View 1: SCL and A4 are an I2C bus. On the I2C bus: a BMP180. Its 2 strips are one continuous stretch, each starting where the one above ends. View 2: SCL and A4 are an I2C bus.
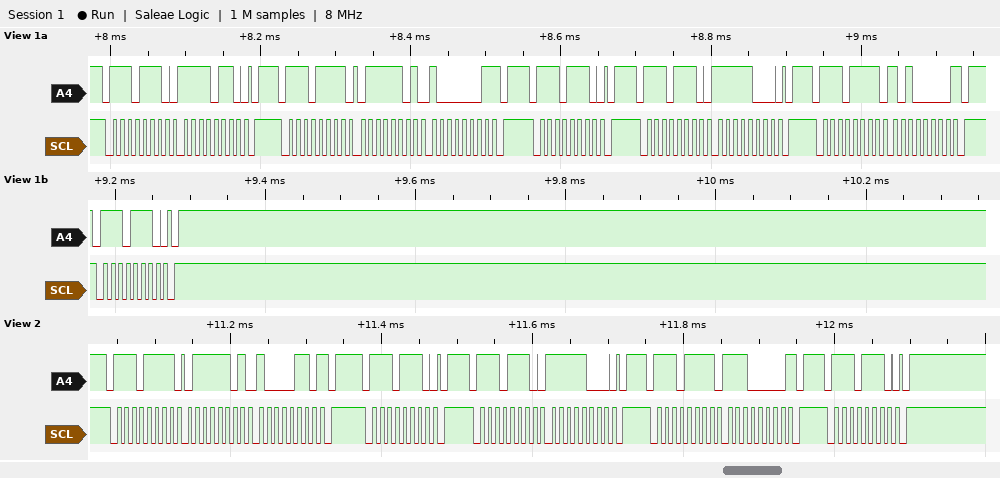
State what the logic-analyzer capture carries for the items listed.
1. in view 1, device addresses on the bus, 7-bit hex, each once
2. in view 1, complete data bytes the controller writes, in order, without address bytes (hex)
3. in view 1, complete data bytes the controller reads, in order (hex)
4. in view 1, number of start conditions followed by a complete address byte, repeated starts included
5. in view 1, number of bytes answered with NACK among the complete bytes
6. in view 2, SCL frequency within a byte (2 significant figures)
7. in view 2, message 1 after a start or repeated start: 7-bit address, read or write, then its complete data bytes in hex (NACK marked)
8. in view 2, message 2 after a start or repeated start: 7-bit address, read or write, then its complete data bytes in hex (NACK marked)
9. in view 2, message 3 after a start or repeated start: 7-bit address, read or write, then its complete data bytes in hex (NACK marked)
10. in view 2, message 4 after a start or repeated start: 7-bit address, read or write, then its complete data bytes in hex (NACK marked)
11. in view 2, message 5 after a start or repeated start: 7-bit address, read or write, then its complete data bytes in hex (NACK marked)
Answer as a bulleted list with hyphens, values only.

- 0x77
- F6 F8
- 7D 81 A0
- 6
- 2
- 100 kHz
- 0x77 read: 7D 86 NACK
- 0x77 write
- 0x77 write: F8
- 0x77 read: E0 NACK
- 0x77 write
